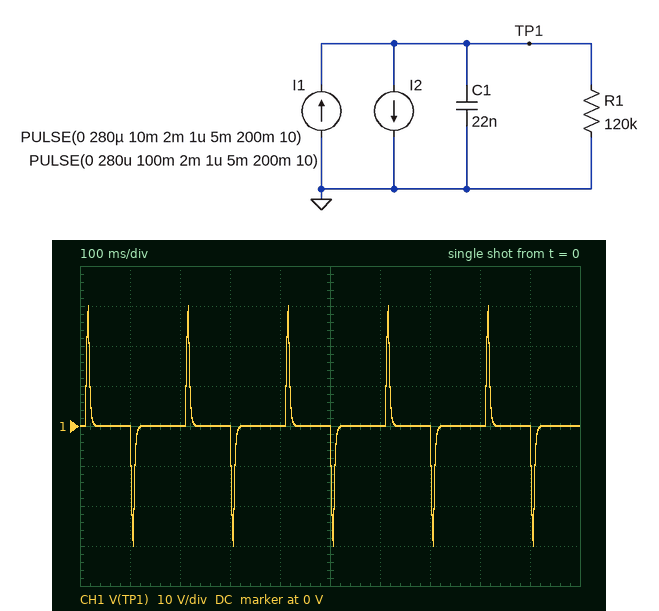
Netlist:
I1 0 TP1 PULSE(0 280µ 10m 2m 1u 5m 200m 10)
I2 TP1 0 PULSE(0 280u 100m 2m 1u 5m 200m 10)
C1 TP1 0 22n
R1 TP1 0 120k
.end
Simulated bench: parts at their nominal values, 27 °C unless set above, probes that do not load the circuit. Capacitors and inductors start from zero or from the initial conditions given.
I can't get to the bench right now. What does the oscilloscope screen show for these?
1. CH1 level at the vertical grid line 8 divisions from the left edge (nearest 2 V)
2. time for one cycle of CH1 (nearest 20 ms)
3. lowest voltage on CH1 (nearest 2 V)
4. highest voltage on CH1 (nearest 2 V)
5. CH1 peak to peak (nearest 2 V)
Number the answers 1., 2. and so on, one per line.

1. 0 V
2. 200 ms
3. -30 V
4. 30 V
5. 60 V
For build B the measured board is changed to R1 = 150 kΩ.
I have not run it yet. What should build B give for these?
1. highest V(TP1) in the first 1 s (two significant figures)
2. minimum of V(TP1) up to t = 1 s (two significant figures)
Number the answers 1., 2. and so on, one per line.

1. 35 V
2. -35 V
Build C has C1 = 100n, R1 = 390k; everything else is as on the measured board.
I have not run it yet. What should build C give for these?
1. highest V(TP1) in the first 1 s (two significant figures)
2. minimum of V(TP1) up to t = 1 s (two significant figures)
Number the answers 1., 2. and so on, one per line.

1. 16 V
2. -14 V
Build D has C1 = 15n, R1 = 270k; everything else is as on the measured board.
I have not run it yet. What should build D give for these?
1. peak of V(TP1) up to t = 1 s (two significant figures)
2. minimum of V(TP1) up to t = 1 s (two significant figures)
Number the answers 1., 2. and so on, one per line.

1. 58 V
2. -58 V
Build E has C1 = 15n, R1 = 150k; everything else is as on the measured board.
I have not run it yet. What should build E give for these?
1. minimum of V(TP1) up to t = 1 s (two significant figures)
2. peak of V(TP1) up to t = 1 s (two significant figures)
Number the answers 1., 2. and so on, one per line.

1. -39 V
2. 39 V
